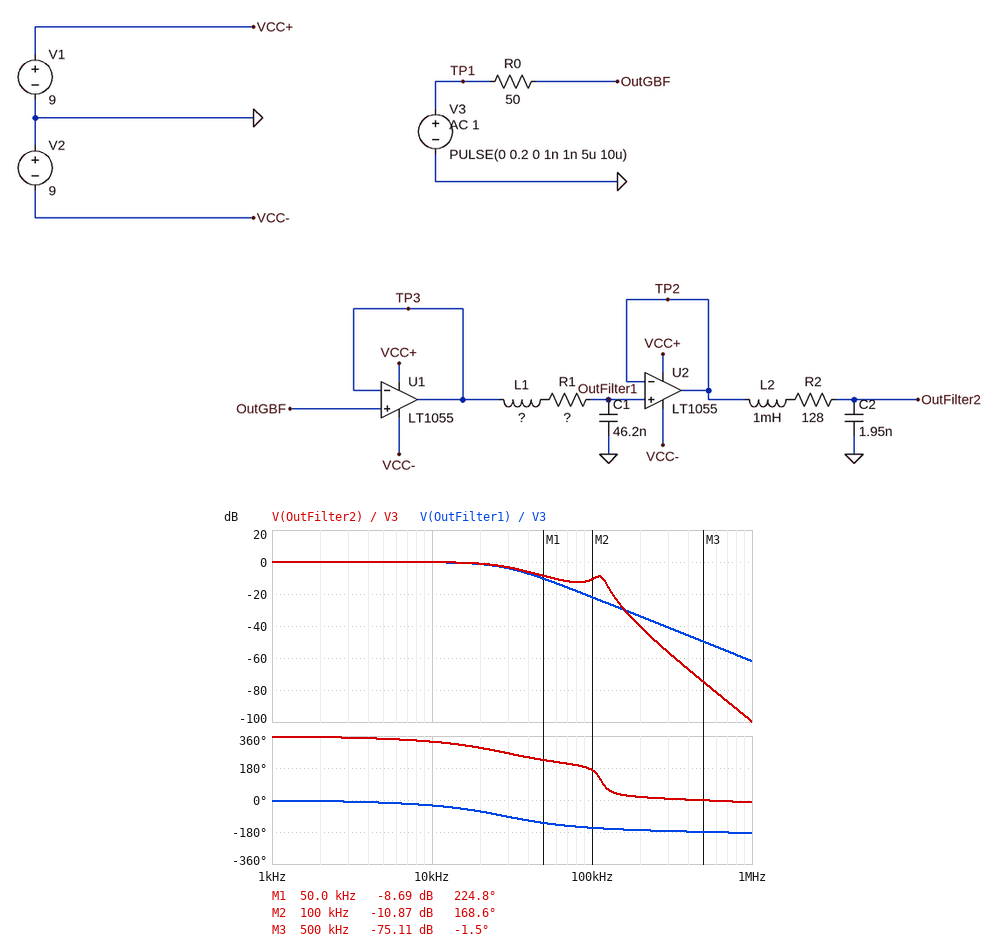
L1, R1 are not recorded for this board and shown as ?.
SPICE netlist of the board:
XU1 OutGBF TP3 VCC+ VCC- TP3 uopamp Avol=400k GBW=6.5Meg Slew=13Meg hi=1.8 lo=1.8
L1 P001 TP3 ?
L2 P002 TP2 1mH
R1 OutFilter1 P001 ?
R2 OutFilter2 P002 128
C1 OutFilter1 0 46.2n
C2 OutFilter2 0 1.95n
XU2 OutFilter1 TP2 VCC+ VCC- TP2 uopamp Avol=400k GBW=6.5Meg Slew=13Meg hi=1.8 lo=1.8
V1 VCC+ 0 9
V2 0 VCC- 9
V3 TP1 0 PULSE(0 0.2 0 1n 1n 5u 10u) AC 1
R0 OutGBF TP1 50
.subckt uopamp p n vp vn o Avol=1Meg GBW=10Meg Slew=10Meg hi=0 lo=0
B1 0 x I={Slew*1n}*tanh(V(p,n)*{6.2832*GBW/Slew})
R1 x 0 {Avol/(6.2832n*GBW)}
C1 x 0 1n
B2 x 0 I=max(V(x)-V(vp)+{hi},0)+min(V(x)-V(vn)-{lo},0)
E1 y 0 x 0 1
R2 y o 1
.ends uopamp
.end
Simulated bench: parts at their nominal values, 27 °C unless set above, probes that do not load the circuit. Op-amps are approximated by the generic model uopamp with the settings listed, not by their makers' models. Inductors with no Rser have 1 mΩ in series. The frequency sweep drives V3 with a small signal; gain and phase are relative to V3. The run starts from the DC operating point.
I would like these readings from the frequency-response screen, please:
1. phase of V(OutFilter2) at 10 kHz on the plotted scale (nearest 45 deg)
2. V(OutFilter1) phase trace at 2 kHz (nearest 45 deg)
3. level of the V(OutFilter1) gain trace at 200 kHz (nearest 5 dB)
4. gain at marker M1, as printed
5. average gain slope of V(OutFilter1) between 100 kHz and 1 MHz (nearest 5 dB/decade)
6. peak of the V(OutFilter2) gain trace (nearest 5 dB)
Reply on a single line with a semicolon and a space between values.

315 deg; 0 deg; -35 dB; -8.69 dB; -40 dB/decade; 0 dB
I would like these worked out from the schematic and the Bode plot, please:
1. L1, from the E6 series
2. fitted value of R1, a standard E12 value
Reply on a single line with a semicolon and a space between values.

680 µH; 180 Ω
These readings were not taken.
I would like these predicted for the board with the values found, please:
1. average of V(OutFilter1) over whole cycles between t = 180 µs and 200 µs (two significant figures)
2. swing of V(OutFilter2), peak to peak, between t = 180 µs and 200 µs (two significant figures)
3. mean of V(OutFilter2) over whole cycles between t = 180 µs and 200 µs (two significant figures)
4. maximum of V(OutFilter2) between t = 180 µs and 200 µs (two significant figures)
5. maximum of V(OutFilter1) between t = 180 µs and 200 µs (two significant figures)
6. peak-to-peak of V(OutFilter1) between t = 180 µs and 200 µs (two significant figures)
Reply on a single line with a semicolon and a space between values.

100 mV; 73 mV; 100 mV; 140 mV; 110 mV; 20 mV
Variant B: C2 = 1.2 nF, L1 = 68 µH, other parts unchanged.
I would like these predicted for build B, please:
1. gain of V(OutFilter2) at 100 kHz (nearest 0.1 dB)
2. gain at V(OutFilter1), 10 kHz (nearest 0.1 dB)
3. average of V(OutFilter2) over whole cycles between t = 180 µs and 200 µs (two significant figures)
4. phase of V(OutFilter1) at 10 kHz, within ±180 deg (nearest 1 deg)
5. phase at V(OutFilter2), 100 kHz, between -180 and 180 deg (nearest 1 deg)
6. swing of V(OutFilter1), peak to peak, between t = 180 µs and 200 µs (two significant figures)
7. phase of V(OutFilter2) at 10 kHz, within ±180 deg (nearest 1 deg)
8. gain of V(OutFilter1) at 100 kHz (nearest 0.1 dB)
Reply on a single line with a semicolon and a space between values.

-8.9 dB; -1.0 dB; 100 mV; -28 deg; -105 deg; 55 mV; -29 deg; -14.4 dB
